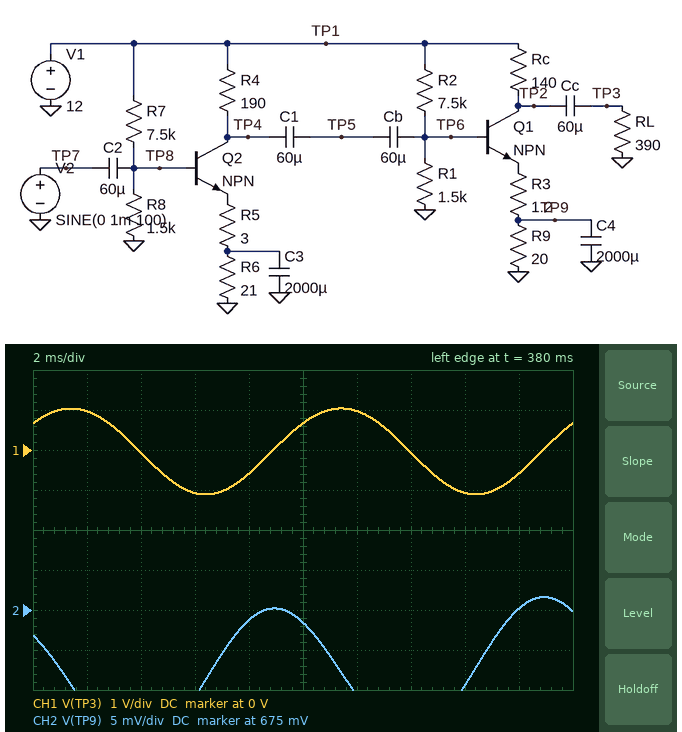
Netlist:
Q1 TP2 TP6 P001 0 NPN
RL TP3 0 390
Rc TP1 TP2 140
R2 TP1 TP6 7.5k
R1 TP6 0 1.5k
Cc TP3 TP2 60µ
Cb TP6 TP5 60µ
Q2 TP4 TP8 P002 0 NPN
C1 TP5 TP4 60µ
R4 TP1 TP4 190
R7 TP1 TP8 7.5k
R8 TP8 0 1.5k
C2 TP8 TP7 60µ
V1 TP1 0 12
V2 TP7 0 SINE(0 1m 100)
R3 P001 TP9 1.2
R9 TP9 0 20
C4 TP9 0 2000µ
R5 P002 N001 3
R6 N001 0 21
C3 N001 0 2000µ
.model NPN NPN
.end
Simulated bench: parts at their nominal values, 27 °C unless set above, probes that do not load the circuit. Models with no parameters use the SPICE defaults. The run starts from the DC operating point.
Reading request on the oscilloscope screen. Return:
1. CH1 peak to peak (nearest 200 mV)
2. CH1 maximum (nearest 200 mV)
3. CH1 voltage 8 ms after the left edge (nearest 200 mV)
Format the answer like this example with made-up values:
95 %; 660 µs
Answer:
2.2 V; 1.0 V; -600 mV
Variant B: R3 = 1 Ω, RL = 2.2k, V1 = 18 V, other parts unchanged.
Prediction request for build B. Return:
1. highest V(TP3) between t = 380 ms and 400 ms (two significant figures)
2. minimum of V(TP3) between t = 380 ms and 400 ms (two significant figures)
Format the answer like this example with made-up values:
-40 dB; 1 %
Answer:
1.6 V; -1.9 V
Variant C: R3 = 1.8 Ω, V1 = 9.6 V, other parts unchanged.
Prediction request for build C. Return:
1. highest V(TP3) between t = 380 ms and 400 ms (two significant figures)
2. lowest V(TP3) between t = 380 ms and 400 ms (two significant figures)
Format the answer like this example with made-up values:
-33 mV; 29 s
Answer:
740 mV; -810 mV
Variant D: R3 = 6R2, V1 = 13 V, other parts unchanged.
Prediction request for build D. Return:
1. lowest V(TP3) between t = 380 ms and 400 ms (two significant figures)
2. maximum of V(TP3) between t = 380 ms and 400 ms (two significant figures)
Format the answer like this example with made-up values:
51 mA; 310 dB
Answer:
-510 mV; 470 mV
